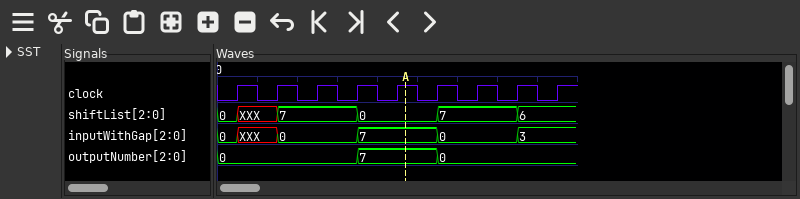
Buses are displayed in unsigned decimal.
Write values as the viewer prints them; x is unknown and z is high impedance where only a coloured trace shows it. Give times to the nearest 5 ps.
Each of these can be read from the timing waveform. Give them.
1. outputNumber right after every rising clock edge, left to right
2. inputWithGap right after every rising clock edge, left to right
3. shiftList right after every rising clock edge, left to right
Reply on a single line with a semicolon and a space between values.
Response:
0, 0, 0, 7, 7, 0, 0, 0, 0; XXX, 0, 0, 7, 7, 0, 0, 3, 3; XXX, 7, 7, 0, 0, 7, 7, 6, 6
